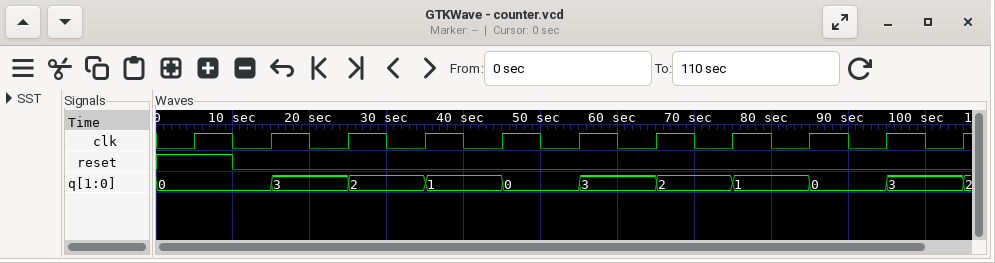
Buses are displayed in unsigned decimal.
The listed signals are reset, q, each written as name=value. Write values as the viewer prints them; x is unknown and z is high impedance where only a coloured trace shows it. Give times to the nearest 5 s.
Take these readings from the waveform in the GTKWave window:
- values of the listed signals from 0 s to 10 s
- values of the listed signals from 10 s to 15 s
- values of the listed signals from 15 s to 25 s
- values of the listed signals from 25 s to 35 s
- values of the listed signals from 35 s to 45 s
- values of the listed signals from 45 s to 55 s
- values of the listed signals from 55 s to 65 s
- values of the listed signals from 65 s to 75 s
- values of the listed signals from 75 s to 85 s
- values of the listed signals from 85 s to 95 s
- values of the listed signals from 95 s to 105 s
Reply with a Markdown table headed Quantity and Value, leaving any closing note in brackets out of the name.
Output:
| Quantity | Value |
|---|---|
| values of the listed signals from 0 s to 10 s | reset=1, q=0 |
| values of the listed signals from 10 s to 15 s | reset=0, q=0 |
| values of the listed signals from 15 s to 25 s | reset=0, q=3 |
| values of the listed signals from 25 s to 35 s | reset=0, q=2 |
| values of the listed signals from 35 s to 45 s | reset=0, q=1 |
| values of the listed signals from 45 s to 55 s | reset=0, q=0 |
| values of the listed signals from 55 s to 65 s | reset=0, q=3 |
| values of the listed signals from 65 s to 75 s | reset=0, q=2 |
| values of the listed signals from 75 s to 85 s | reset=0, q=1 |
| values of the listed signals from 85 s to 95 s | reset=0, q=0 |
| values of the listed signals from 95 s to 105 s | reset=0, q=3 |
